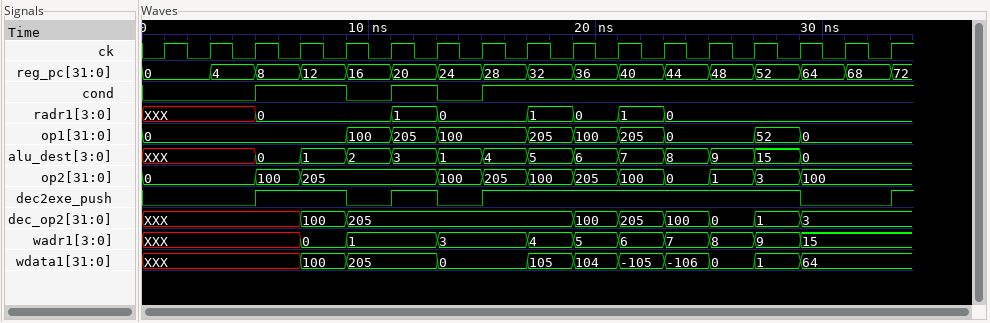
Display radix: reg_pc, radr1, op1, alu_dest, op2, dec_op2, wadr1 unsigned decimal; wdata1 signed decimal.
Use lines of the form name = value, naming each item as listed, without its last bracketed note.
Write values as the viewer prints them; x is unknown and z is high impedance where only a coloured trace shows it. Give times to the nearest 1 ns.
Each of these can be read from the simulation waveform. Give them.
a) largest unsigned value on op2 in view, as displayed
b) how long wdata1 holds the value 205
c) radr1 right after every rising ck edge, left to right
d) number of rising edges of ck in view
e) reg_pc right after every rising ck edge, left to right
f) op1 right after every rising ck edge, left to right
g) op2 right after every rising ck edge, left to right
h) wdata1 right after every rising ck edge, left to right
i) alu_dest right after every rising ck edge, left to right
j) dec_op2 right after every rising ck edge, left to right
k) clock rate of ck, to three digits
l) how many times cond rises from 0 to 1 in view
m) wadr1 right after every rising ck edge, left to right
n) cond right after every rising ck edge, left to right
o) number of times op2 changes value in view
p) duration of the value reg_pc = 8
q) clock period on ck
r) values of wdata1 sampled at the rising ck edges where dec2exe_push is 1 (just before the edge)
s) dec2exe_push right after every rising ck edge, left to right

largest unsigned value on op2 in view, as displayed = 205
how long wdata1 holds the value 205 = 4 ns
radr1 right after every rising ck edge, left to right = XXX, XXX, 0, 0, 0, 1, 0, 0, 1, 0, 1, 0, 0, 0, 0, 0, 0
number of rising edges of ck in view = 17
reg_pc right after every rising ck edge, left to right = 0, 4, 8, 12, 16, 20, 24, 28, 32, 36, 40, 44, 48, 52, 64, 68, 72
op1 right after every rising ck edge, left to right = 0, 0, 0, 0, 100, 205, 100, 100, 205, 100, 205, 0, 0, 52, 0, 0, 0
op2 right after every rising ck edge, left to right = 0, 0, 100, 205, 205, 205, 100, 205, 100, 205, 100, 0, 1, 3, 100, 100, 100
wdata1 right after every rising ck edge, left to right = XXX, XXX, XXX, 100, 205, 205, 0, 0, 105, 104, -105, -106, 0, 1, 64, 64, 64
alu_dest right after every rising ck edge, left to right = XXX, XXX, 0, 1, 2, 3, 1, 4, 5, 6, 7, 8, 9, 15, 0, 0, 0
dec_op2 right after every rising ck edge, left to right = XXX, XXX, XXX, 100, 205, 205, 205, 205, 205, 100, 205, 100, 0, 1, 3, 3, 3
clock rate of ck, to three digits = 500 MHz
how many times cond rises from 0 to 1 in view = 3
wadr1 right after every rising ck edge, left to right = XXX, XXX, XXX, 0, 1, 1, 3, 3, 4, 5, 6, 7, 8, 9, 15, 15, 15
cond right after every rising ck edge, left to right = 0 0 1 1 0 1 0 1 1 1 1 1 1 1 1 1 1
number of times op2 changes value in view = 11
duration of the value reg_pc = 8 = 2 ns
clock period on ck = 2 ns
values of wdata1 sampled at the rising ck edges where dec2exe_push is 1 = XXX, 100, 205, 0, 105, 104, -105, -106, 0, 1
dec2exe_push right after every rising ck edge, left to right = 0 0 1 1 0 1 0 1 1 1 1 1 1 1 0 0 1
